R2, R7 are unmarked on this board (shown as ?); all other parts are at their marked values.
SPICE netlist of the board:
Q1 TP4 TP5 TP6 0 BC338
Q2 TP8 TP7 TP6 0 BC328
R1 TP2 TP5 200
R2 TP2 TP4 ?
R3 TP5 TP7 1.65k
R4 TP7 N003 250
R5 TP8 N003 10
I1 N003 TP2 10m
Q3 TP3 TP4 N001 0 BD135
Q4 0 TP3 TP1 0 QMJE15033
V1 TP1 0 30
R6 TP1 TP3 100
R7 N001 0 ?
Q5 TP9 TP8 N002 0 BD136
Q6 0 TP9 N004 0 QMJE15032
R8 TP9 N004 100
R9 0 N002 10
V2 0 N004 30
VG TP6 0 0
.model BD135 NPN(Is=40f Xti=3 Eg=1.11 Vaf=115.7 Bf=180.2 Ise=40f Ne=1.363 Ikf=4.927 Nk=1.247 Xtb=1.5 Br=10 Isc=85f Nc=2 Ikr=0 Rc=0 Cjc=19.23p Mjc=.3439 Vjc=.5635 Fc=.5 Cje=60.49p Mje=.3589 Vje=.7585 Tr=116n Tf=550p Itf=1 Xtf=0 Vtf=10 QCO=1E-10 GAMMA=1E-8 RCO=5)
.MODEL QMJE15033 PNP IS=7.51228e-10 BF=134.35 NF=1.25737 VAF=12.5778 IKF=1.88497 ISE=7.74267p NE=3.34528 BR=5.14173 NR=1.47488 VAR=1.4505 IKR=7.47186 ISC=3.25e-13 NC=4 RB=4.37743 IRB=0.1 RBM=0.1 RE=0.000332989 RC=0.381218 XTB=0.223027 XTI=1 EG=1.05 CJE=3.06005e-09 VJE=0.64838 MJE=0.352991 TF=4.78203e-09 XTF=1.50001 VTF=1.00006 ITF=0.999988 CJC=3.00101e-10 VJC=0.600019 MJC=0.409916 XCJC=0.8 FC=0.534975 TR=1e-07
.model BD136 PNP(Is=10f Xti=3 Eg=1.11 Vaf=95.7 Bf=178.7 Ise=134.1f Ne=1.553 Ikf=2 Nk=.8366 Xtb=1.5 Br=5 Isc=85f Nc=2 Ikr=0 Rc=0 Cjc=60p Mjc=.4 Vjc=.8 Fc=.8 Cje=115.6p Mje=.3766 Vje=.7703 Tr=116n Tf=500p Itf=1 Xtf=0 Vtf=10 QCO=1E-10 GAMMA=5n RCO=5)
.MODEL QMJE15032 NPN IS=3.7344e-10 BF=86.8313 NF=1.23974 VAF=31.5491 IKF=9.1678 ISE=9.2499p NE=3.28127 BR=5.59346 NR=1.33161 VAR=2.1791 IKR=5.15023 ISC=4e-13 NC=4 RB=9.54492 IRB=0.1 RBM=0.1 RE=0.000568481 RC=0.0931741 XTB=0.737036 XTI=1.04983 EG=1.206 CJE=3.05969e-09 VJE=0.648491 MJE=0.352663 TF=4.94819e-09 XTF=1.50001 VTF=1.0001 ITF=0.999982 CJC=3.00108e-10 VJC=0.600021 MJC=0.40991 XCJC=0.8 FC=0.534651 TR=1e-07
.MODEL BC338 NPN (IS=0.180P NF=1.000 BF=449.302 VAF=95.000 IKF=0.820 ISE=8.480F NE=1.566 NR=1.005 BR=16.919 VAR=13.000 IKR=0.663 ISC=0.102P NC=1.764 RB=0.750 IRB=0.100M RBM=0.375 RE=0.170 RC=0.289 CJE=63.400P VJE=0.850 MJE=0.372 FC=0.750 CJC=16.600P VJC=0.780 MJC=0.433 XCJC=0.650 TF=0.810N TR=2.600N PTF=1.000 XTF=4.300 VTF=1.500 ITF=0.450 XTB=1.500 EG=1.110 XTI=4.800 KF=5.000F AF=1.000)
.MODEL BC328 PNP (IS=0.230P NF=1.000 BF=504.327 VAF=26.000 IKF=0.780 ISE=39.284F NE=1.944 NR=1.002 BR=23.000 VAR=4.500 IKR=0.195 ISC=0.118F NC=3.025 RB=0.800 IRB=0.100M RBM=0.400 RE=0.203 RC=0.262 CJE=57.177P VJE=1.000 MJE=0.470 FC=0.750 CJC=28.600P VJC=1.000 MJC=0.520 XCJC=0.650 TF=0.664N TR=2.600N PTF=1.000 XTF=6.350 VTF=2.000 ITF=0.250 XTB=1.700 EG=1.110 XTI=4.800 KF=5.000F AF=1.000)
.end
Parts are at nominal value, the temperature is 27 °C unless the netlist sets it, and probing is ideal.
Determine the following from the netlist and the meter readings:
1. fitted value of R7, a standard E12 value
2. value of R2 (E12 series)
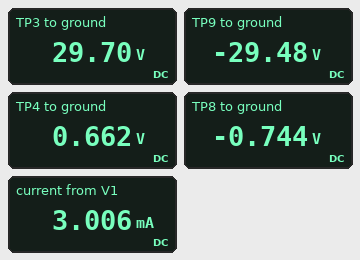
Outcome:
6.8 Ω
15 Ω
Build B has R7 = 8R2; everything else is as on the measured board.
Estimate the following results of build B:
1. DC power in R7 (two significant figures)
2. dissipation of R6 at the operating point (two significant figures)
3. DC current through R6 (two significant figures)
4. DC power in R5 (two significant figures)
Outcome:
62 µW
750 µW
2.7 mA
850 µW
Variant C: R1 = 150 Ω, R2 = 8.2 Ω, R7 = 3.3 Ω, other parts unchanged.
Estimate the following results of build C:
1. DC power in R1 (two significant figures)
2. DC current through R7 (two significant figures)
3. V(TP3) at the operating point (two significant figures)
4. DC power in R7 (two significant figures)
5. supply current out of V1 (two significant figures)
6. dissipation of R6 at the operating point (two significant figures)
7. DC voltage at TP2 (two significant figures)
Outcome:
95 µW
6.7 mA
29 V
150 µW
240 mA
3.7 mW
760 mV
